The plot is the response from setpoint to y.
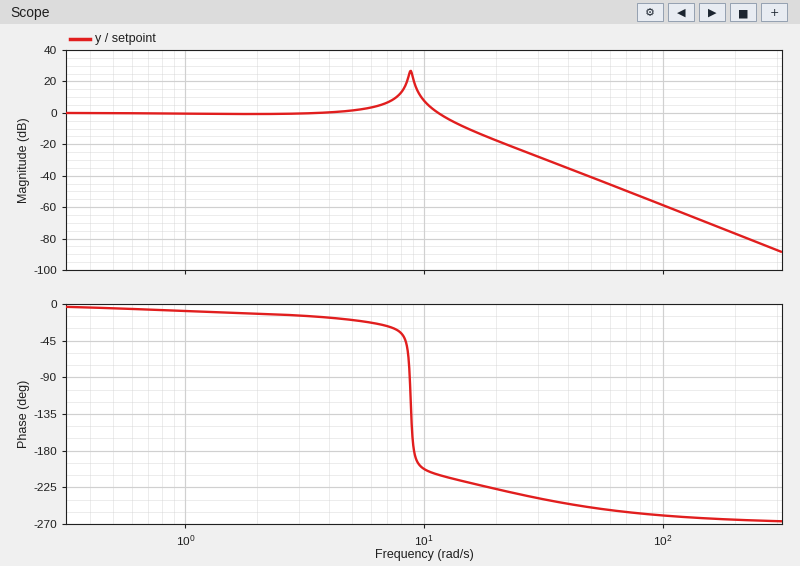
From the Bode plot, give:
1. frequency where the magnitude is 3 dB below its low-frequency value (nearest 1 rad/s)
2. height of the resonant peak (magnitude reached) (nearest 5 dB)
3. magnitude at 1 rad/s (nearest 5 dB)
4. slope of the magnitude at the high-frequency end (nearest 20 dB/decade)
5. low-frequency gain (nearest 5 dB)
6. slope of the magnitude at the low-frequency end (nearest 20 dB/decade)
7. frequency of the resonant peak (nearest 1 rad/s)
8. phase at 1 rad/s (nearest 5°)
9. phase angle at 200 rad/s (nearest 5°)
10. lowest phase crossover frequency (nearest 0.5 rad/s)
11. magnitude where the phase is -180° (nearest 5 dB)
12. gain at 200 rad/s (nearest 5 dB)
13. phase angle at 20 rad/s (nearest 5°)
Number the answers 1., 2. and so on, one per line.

1. 12 rad/s
2. 25 dB
3. 0 dB
4. -60 dB/decade
5. 0 dB
6. 0 dB/decade
7. 9 rad/s
8. -10°
9. -265°
10. 9.0 rad/s
11. 20 dB
12. -75 dB
13. -225°
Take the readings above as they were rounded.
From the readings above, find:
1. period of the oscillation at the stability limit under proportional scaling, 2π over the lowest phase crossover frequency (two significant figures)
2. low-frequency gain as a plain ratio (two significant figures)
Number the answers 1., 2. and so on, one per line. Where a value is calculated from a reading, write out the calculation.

1. 2π / 9 = 0.70 s
2. 10^(0 / 20) = 1.0
